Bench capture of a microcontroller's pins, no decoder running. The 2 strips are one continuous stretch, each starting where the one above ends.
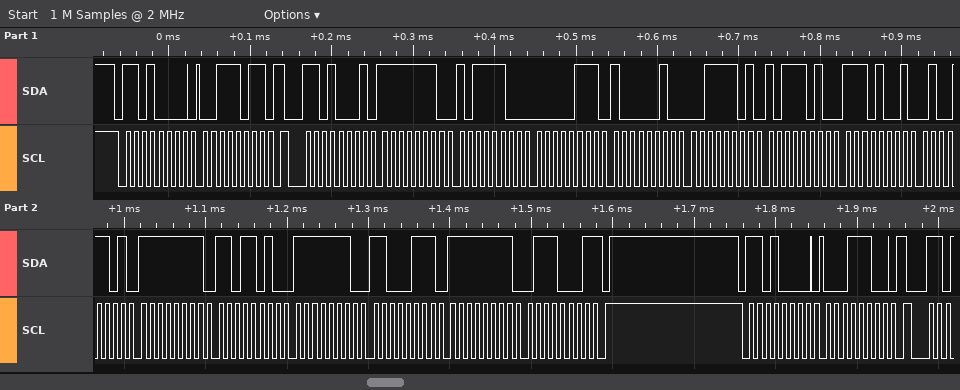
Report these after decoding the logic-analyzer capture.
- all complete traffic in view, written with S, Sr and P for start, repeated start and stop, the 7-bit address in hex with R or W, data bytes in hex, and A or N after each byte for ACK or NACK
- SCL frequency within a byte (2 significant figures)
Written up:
S 68W A 3B A Sr 68R A FE A BC A 07 A 82 A 3D A BA A E9 A 4D A FF A DA A FE A C7 A FF A 71 N P S 68W A 1C A
100 kHz
